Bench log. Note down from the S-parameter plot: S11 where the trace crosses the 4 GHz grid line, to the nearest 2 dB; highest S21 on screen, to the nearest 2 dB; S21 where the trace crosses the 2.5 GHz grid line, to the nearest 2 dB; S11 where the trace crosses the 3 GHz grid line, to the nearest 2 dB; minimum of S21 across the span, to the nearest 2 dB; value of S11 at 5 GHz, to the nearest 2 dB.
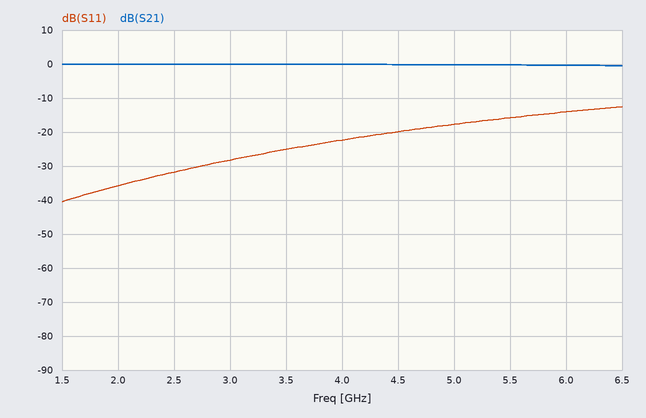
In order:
-22 dB
0 dB
0 dB
-28 dB
0 dB
-18 dB
